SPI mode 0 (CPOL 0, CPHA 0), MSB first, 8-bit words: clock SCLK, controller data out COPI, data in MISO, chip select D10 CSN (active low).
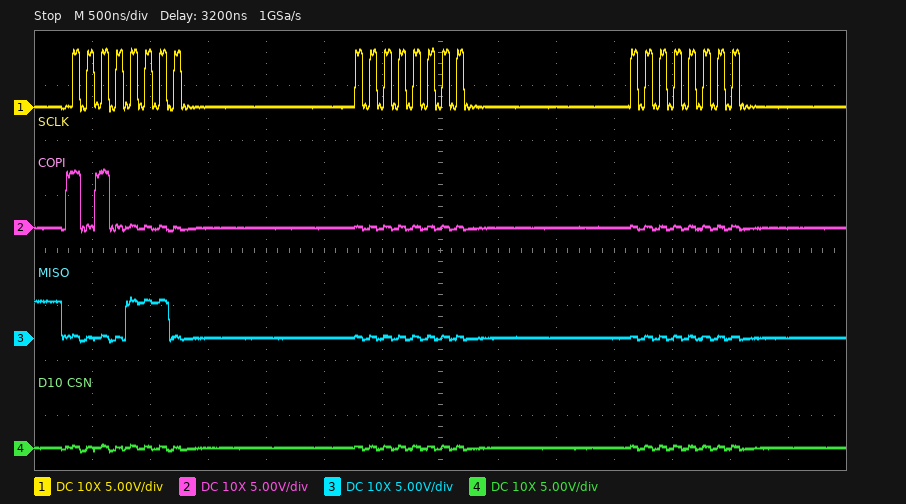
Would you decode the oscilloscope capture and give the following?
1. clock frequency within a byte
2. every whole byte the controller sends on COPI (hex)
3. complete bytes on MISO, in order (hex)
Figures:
8 MHz
0xA0 0x00 0x00
0x0E 0x00 0x00
